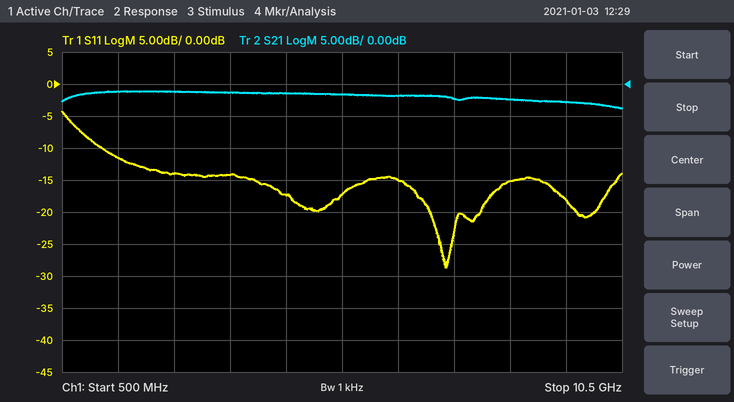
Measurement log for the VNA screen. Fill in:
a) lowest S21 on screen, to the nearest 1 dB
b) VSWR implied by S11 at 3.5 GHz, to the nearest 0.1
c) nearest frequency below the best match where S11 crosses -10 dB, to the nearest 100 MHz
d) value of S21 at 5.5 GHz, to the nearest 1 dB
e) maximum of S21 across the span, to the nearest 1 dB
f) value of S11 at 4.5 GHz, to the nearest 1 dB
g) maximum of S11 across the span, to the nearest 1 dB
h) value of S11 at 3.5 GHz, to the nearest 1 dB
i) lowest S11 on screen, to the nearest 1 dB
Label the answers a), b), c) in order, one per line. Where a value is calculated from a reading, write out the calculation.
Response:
a) -4 dB
b) |Γ| = 10^(-14/20) = 0.1995; VSWR = (1 + 0.1995)/(1 − 0.1995) ≈ 1.5
c) 1.2 GHz
d) -2 dB
e) -1 dB
f) -17 dB
g) -4 dB
h) -14 dB
i) -29 dB
